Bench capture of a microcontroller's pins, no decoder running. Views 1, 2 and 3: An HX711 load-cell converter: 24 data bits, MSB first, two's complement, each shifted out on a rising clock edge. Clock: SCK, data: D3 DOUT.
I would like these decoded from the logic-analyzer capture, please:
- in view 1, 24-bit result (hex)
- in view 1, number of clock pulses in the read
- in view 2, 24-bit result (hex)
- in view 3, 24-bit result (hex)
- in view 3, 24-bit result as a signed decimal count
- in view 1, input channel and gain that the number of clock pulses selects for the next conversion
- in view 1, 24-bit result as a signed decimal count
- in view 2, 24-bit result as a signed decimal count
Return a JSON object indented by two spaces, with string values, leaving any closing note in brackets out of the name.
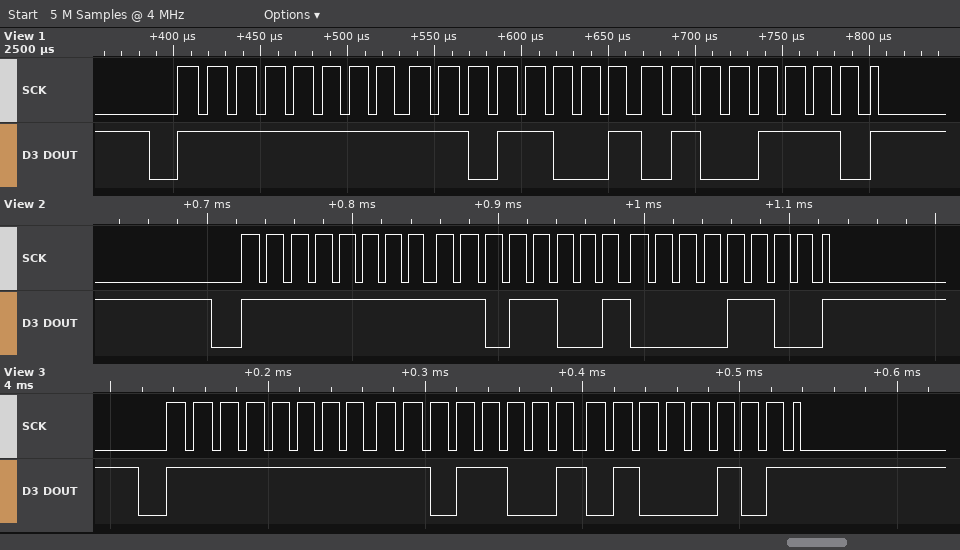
{
  "in view 1, 24-bit result": "0xFFD94E",
  "in view 1, number of clock pulses in the read": "25",
  "in view 2, 24-bit result": "0xFFD90C",
  "in view 3, 24-bit result": "0xFFD945",
  "in view 3, 24-bit result as a signed decimal count": "-9915",
  "in view 1, input channel and gain that the number of clock pulses selects for the next conversion": "channel A, gain 128",
  "in view 1, 24-bit result as a signed decimal count": "-9906",
  "in view 2, 24-bit result as a signed decimal count": "-9972"
}
